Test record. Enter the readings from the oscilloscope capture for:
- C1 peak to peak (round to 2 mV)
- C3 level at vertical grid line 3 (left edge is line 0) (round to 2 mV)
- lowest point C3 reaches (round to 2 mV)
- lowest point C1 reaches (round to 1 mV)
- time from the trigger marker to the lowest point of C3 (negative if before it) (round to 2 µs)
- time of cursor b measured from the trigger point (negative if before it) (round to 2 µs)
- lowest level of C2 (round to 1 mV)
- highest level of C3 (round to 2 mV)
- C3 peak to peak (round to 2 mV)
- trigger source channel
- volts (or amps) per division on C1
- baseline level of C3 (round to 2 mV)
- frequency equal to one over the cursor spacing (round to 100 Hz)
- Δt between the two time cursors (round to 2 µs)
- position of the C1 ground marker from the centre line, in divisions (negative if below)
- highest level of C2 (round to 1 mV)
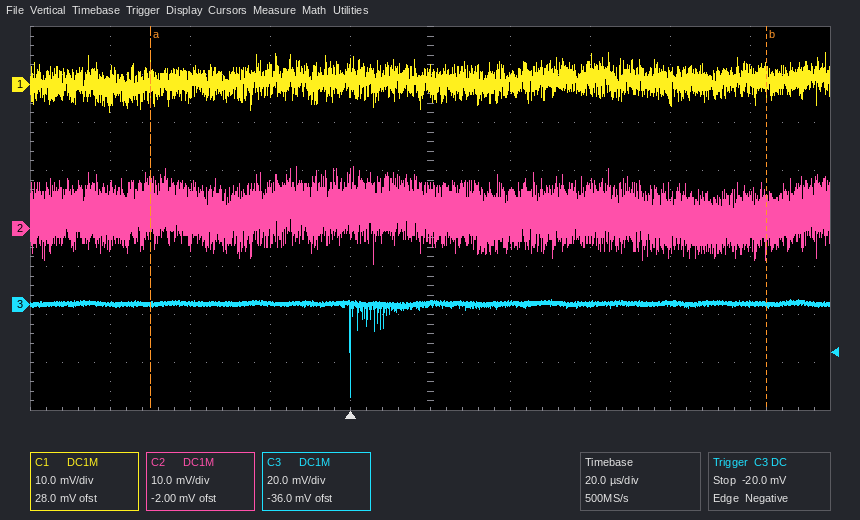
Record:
12 mV
0 mV
-38 mV
-6 mV
0 µs
+104 µs
-8 mV
2 mV
40 mV
C3
10 mV
0 mV
6.5 kHz
154 µs
+2.8 div
13 mV
